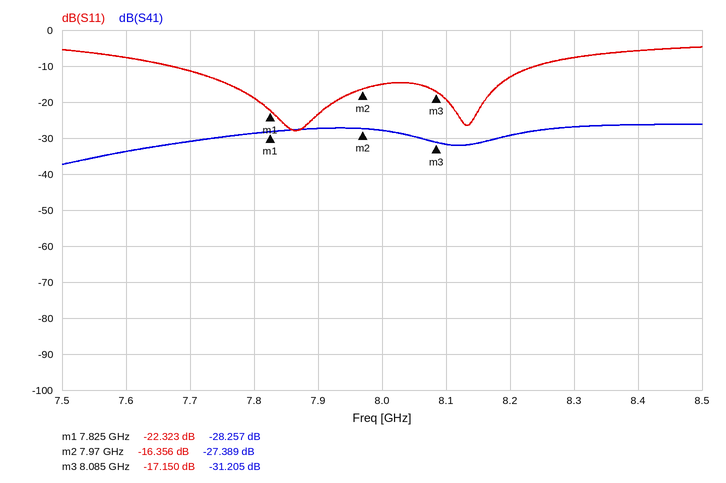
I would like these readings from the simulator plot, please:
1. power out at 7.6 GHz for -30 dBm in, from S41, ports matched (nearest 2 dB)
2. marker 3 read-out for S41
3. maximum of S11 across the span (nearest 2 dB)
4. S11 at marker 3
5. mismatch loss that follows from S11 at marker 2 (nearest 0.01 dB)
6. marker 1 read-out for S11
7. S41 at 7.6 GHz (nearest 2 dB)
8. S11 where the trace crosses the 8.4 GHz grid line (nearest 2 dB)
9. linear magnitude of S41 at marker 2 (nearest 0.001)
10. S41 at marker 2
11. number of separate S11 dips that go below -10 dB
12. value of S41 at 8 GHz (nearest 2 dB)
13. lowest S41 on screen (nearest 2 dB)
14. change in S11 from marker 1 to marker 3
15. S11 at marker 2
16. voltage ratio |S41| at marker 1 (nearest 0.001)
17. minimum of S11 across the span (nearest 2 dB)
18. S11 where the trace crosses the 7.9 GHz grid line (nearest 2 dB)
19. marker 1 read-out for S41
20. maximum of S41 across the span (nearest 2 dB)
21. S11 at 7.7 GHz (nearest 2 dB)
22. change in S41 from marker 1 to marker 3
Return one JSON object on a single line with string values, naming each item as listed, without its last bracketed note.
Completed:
{"power out at 7.6 GHz for -30 dBm in, from S41, ports matched": "-64 dBm", "marker 3 read-out for S41": "-31.205 dB", "maximum of S11 across the span": "-4 dB", "S11 at marker 3": "-17.150 dB", "mismatch loss that follows from S11 at marker 2": "0.10 dB", "marker 1 read-out for S11": "-22.323 dB", "S41 at 7.6 GHz": "-34 dB", "S11 where the trace crosses the 8.4 GHz grid line": "-6 dB", "linear magnitude of S41 at marker 2": "0.043", "S41 at marker 2": "-27.389 dB", "number of separate S11 dips that go below -10 dB": "2", "value of S41 at 8 GHz": "-28 dB", "lowest S41 on screen": "-38 dB", "change in S11 from marker 1 to marker 3": "5.173 dB", "S11 at marker 2": "-16.356 dB", "voltage ratio |S41| at marker 1": "0.039", "minimum of S11 across the span": "-28 dB", "S11 where the trace crosses the 7.9 GHz grid line": "-24 dB", "marker 1 read-out for S41": "-28.257 dB", "maximum of S41 across the span": "-26 dB", "S11 at 7.7 GHz": "-12 dB", "change in S41 from marker 1 to marker 3": "-2.948 dB"}
